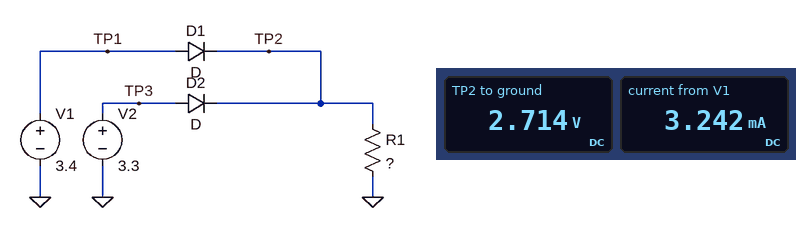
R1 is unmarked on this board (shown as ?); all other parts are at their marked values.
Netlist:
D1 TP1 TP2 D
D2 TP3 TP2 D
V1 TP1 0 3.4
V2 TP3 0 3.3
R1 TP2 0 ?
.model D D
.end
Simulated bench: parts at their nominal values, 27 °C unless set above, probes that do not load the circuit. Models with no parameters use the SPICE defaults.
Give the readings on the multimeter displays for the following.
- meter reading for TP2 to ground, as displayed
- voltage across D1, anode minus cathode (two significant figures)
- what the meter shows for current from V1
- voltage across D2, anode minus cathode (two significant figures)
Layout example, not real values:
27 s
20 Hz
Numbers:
2.714 V
690 mV
3.242 mA
590 mV
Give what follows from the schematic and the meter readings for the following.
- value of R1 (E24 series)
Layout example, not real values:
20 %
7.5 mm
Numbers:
820 Ω
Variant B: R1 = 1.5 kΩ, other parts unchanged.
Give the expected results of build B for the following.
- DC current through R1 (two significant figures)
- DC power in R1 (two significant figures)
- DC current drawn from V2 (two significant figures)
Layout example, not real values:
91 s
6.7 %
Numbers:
1.8 mA
5.0 mW
37 µA
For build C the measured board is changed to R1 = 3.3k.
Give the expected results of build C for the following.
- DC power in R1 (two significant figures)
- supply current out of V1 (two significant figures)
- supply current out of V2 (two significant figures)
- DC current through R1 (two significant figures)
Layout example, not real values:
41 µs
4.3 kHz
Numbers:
2.3 mW
820 µA
17 µA
830 µA
